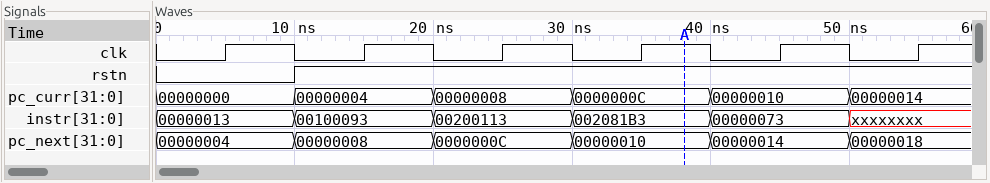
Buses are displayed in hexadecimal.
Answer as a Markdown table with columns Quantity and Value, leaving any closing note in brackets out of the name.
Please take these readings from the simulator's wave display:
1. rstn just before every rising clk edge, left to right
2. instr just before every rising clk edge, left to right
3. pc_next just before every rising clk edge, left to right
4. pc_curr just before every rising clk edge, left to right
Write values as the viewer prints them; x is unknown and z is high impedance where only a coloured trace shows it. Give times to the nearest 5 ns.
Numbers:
| Quantity | Value |
|---|---|
| rstn just before every rising clk edge, left to right | 0 1 1 1 1 1 |
| instr just before every rising clk edge, left to right | 00000013, 00100093, 00200113, 002081B3, 00000073, xxxxxxxx |
| pc_next just before every rising clk edge, left to right | 00000004, 00000008, 0000000C, 00000010, 00000014, 00000018 |
| pc_curr just before every rising clk edge, left to right | 00000000, 00000004, 00000008, 0000000C, 00000010, 00000014 |
